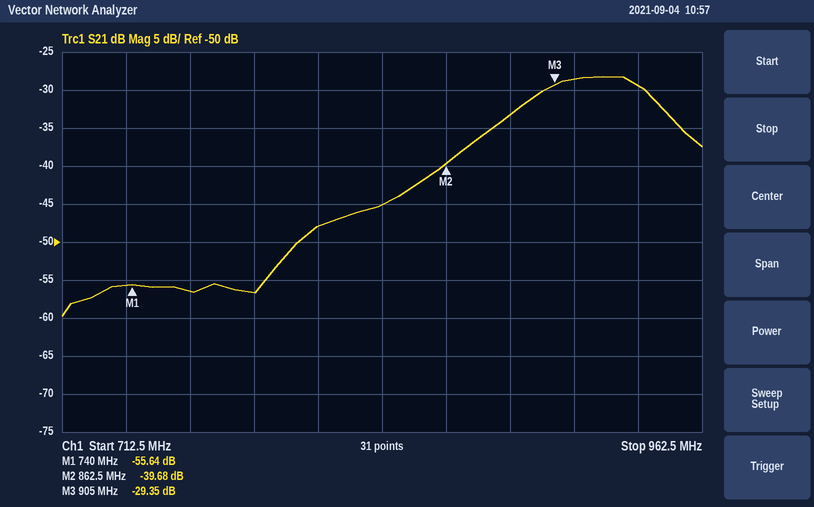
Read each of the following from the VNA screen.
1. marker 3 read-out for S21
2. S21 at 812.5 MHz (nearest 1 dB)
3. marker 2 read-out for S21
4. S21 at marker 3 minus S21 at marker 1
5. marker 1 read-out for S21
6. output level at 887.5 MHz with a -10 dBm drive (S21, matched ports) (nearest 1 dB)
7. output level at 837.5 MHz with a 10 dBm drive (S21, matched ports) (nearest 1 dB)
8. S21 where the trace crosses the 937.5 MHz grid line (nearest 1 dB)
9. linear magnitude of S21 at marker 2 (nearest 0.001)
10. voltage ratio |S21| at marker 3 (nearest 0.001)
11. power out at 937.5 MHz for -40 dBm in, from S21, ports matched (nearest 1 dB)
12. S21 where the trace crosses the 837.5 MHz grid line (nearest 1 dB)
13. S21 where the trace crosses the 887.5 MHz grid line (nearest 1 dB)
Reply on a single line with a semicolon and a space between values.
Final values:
-29.35 dB; -48 dB; -39.68 dB; 26.29 dB; -55.64 dB; -43 dBm; -35 dBm; -29 dB; 0.010; 0.034; -69 dBm; -45 dB; -33 dB
